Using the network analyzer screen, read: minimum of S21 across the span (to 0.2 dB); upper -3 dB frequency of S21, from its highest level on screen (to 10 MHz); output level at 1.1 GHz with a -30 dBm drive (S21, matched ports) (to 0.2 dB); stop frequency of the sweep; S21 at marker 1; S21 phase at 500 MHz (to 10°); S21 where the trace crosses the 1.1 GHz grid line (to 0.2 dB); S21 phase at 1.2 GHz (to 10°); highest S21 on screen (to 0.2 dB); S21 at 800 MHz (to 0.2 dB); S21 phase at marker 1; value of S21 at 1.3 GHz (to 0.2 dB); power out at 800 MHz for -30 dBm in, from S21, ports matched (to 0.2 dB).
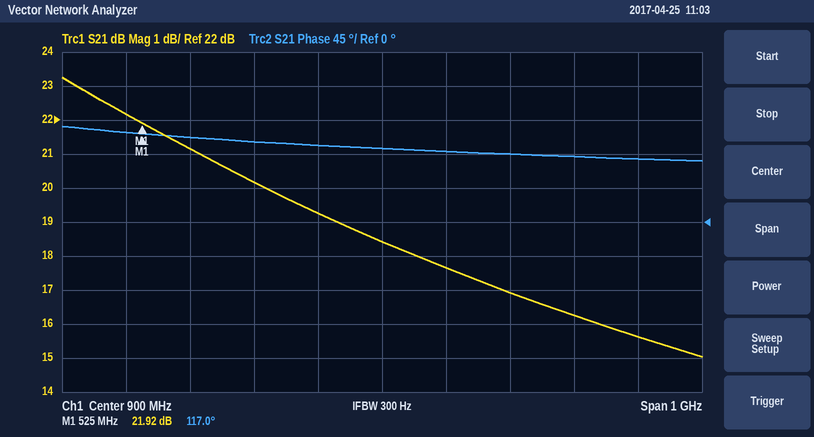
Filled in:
15.0 dB
690 MHz
-13.0 dBm
1.4 GHz
21.92 dB
120°
17.0 dB
90°
23.2 dB
19.2 dB
117.0°
15.6 dB
-10.8 dBm
